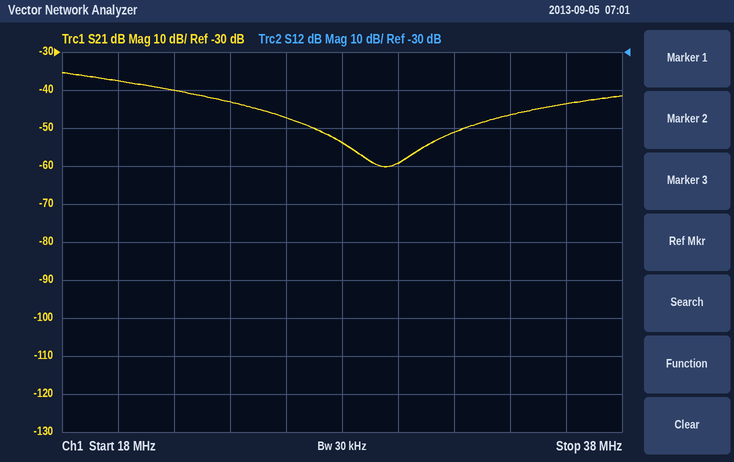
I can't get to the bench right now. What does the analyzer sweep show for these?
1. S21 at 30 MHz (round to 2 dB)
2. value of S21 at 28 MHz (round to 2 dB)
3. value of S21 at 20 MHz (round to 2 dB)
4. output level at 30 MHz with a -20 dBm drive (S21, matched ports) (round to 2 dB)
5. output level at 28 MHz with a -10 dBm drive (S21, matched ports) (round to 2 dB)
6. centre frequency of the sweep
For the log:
-60 dB
-54 dB
-38 dB
-80 dBm
-64 dBm
28 MHz
